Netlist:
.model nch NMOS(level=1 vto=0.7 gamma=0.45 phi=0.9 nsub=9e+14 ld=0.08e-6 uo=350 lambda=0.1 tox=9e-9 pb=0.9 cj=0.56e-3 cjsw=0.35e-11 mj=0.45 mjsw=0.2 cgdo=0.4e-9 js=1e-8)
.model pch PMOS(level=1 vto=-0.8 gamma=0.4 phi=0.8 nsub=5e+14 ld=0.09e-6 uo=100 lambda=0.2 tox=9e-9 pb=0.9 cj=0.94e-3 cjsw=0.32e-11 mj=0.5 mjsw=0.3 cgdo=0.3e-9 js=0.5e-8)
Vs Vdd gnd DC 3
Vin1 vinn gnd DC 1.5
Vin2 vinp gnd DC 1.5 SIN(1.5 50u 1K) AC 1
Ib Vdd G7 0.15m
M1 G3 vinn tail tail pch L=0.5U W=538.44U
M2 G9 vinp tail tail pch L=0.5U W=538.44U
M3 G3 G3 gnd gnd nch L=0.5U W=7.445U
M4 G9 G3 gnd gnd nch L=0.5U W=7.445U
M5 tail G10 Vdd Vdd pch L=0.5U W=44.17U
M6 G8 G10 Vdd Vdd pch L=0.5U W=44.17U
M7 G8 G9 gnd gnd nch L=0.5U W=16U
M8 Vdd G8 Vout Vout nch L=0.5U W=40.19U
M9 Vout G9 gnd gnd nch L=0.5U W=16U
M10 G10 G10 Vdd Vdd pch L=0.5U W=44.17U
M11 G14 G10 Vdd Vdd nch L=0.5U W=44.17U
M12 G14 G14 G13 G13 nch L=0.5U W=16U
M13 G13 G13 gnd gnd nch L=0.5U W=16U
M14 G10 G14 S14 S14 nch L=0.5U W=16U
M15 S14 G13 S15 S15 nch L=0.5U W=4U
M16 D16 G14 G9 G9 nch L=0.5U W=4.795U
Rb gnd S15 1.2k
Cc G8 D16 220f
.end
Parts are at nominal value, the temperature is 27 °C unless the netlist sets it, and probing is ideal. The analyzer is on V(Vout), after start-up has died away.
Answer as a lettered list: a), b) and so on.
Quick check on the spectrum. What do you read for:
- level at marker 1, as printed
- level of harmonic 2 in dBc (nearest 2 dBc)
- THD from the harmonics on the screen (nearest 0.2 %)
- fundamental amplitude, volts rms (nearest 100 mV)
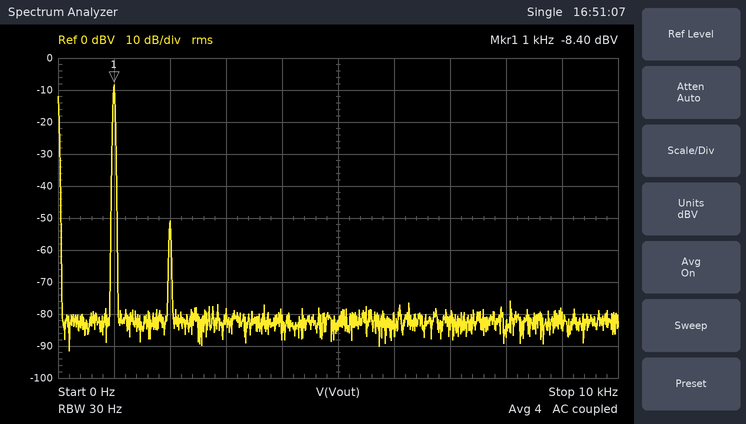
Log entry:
a) -8.40 dBV
b) -42 dBc
c) 0.8 %
d) 400 mV
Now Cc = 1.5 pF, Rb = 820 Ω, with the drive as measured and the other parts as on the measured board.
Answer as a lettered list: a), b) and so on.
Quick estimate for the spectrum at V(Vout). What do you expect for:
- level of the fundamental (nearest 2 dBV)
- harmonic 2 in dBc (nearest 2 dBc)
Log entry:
a) -10 dBV
b) -44 dBc
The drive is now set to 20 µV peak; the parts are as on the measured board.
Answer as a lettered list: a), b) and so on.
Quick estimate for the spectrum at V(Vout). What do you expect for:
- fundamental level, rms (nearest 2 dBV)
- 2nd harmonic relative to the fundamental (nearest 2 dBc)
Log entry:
a) -16 dBV
b) -50 dBc
